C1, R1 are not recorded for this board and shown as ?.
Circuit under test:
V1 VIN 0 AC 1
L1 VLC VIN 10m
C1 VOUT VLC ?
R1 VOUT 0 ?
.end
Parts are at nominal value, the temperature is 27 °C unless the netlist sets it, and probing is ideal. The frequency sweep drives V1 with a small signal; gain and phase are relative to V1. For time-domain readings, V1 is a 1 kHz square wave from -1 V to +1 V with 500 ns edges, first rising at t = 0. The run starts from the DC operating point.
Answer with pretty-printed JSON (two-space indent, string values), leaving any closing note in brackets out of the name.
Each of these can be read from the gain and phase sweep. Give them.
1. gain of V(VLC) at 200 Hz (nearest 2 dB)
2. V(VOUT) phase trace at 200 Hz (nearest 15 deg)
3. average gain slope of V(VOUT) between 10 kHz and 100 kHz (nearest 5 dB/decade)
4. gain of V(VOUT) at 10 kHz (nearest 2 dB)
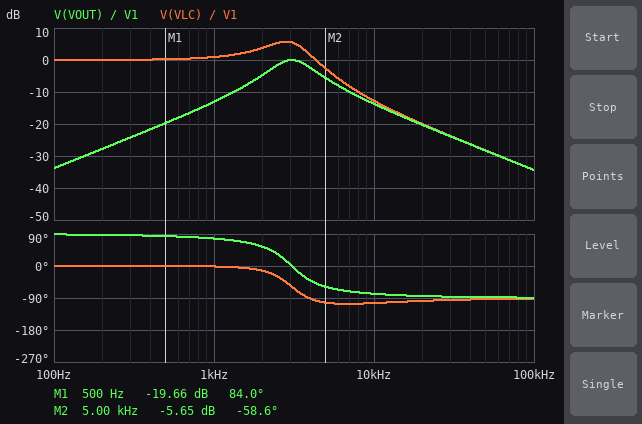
{
  "gain of V(VLC) at 200 Hz": "0 dB",
  "V(VOUT) phase trace at 200 Hz": "90 deg",
  "average gain slope of V(VOUT) between 10 kHz and 100 kHz": "-20 dB/decade",
  "gain of V(VOUT) at 10 kHz": "-14 dB"
}
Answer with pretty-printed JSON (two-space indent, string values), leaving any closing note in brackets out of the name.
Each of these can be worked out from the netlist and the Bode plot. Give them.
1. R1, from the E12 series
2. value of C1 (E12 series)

{
  "R1, from the E12 series": "120 Ω",
  "value of C1": "270 nF"
}
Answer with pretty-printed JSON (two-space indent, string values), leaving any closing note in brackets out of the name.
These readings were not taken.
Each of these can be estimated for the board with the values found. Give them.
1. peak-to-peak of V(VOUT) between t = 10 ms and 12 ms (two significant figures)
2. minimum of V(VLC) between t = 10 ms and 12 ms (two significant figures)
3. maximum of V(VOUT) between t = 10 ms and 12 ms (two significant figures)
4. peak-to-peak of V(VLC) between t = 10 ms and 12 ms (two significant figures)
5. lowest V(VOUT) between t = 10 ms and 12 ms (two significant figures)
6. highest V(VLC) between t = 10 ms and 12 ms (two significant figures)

{
  "peak-to-peak of V(VOUT) between t = 10 ms and 12 ms": "1.7 V",
  "minimum of V(VLC) between t = 10 ms and 12 ms": "-1.9 V",
  "maximum of V(VOUT) between t = 10 ms and 12 ms": "860 mV",
  "peak-to-peak of V(VLC) between t = 10 ms and 12 ms": "3.8 V",
  "lowest V(VOUT) between t = 10 ms and 12 ms": "-860 mV",
  "highest V(VLC) between t = 10 ms and 12 ms": "1.9 V"
}
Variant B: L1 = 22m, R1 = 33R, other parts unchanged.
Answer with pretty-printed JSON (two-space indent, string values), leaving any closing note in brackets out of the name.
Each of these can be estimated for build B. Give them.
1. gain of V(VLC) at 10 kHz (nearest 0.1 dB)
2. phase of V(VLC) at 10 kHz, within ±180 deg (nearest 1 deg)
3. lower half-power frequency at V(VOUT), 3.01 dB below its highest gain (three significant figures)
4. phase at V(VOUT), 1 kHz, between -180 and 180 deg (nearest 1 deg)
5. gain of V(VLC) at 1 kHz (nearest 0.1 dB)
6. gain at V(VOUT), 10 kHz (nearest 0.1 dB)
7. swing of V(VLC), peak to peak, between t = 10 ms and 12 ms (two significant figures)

{
  "gain of V(VLC) at 10 kHz": "-25.8 dB",
  "phase of V(VLC) at 10 kHz, within ±180 deg": "-149 deg",
  "lower half-power frequency at V(VOUT), 3.01 dB below its highest gain": "1.95 kHz",
  "phase at V(VOUT), 1 kHz, between -180 and 180 deg": "86 deg",
  "gain of V(VLC) at 1 kHz": "2.3 dB",
  "gain at V(VOUT), 10 kHz": "-32.1 dB",
  "swing of V(VLC), peak to peak, between t = 10 ms and 12 ms": "4.0 V"
}
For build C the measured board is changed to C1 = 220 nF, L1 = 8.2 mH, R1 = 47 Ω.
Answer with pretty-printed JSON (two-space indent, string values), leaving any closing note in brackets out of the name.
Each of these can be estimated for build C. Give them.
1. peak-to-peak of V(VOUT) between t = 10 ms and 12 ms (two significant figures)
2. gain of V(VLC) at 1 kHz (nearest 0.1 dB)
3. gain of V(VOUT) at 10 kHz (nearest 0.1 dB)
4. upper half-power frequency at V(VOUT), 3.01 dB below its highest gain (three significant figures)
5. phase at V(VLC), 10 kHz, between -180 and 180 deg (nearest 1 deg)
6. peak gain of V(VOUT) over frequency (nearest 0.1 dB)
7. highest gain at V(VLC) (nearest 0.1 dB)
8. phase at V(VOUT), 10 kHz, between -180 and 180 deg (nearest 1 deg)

{
  "peak-to-peak of V(VOUT) between t = 10 ms and 12 ms": "710 mV",
  "gain of V(VLC) at 1 kHz": "0.6 dB",
  "gain of V(VOUT) at 10 kHz": "-19.5 dB",
  "upper half-power frequency at V(VOUT), 3.01 dB below its highest gain": "4.23 kHz",
  "phase at V(VLC), 10 kHz, between -180 and 180 deg": "-141 deg",
  "peak gain of V(VOUT) over frequency": "0 dB",
  "highest gain at V(VLC)": "12.6 dB",
  "phase at V(VOUT), 10 kHz, between -180 and 180 deg": "-84 deg"
}
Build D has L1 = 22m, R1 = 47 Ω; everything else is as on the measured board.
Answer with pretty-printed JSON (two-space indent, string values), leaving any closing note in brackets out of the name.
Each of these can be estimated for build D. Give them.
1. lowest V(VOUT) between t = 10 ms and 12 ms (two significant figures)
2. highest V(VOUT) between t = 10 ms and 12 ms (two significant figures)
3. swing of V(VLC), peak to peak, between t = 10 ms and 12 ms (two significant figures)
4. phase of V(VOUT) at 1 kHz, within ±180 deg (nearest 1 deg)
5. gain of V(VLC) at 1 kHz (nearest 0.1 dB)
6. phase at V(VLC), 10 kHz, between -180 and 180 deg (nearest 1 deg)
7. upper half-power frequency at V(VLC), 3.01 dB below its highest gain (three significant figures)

{
  "lowest V(VOUT) between t = 10 ms and 12 ms": "-180 mV",
  "highest V(VOUT) between t = 10 ms and 12 ms": "180 mV",
  "swing of V(VLC), peak to peak, between t = 10 ms and 12 ms": "4.0 V",
  "phase of V(VOUT) at 1 kHz, within ±180 deg": "84 deg",
  "gain of V(VLC) at 1 kHz": "2.3 dB",
  "phase at V(VLC), 10 kHz, between -180 and 180 deg": "-139 deg",
  "upper half-power frequency at V(VLC), 3.01 dB below its highest gain": "2.22 kHz"
}
